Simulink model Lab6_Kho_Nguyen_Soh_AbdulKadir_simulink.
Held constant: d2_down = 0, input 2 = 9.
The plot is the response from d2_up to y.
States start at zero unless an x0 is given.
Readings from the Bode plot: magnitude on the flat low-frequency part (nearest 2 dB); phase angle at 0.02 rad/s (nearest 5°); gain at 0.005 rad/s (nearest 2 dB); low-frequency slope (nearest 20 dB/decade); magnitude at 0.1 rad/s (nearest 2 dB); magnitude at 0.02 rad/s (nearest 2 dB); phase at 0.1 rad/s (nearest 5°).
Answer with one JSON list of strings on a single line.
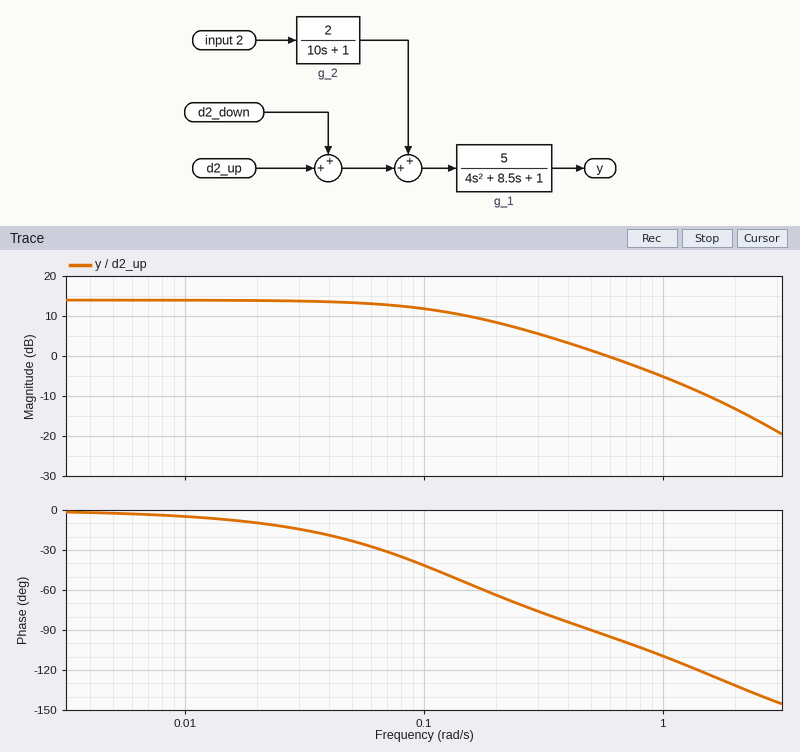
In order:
["14 dB", "-10°", "14 dB", "0 dB/decade", "12 dB", "14 dB", "-40°"]
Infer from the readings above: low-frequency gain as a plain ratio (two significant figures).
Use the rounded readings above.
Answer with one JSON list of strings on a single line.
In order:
["5.0"]
